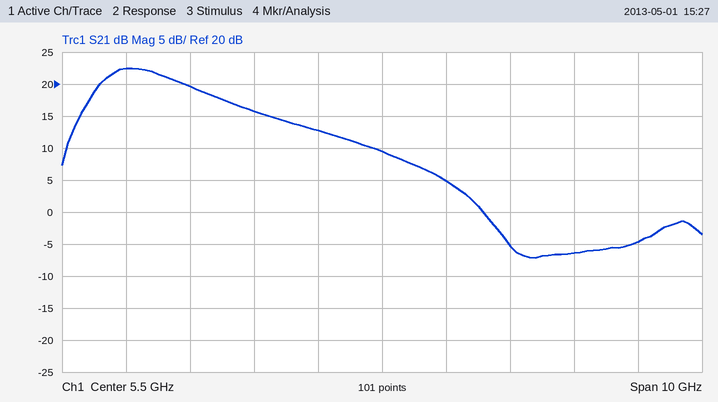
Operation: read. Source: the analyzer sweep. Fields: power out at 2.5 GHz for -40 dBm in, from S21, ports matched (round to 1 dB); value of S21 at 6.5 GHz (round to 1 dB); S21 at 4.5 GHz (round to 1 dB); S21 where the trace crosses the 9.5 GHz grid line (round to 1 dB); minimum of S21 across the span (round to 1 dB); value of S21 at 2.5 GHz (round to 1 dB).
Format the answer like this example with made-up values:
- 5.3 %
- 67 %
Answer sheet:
- -20 dBm
- 5 dB
- 13 dB
- -5 dB
- -7 dB
- 20 dB
